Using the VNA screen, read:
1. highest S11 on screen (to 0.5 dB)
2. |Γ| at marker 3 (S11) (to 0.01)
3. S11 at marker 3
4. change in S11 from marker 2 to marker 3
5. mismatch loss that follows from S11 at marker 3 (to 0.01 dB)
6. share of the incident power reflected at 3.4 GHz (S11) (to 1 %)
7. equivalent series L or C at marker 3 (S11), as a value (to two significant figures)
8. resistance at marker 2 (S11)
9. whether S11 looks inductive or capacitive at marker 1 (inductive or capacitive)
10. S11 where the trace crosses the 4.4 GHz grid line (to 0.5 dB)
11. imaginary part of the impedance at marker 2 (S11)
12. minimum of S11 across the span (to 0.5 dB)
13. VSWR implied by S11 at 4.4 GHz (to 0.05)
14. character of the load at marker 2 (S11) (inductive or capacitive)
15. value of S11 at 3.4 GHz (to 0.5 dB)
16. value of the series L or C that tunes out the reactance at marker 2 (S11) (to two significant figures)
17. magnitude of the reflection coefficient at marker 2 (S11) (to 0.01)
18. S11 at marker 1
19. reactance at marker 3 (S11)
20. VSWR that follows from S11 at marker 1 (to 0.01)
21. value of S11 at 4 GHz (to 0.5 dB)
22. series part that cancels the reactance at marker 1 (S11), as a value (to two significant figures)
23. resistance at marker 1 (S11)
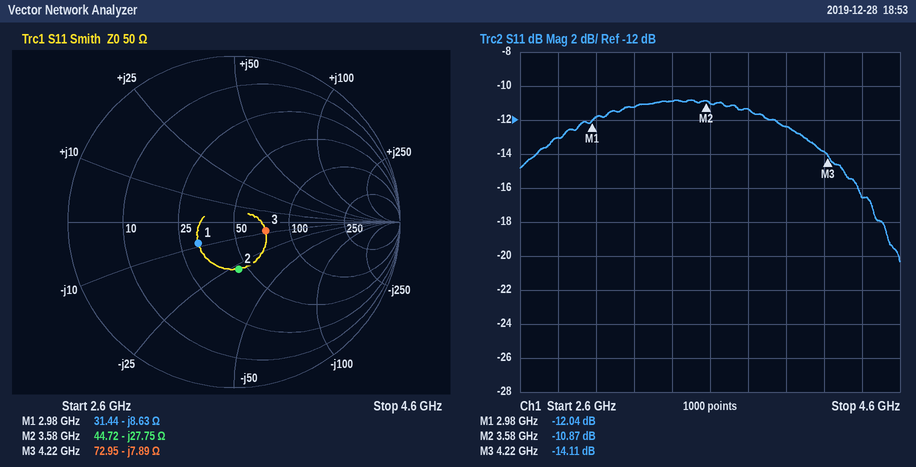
-11.0 dB
0.20
-14.11 dB
-3.24 dB
0.17 dB
8 %
4.8 pF
44.72 Ω
capacitive
-16.5 dB
-27.75 Ω
-20.5 dB
1.35
capacitive
-11.0 dB
1.2 nH
0.29
-12.04 dB
-7.89 Ω
1.67
-12.5 dB
460 pH
31.44 Ω
